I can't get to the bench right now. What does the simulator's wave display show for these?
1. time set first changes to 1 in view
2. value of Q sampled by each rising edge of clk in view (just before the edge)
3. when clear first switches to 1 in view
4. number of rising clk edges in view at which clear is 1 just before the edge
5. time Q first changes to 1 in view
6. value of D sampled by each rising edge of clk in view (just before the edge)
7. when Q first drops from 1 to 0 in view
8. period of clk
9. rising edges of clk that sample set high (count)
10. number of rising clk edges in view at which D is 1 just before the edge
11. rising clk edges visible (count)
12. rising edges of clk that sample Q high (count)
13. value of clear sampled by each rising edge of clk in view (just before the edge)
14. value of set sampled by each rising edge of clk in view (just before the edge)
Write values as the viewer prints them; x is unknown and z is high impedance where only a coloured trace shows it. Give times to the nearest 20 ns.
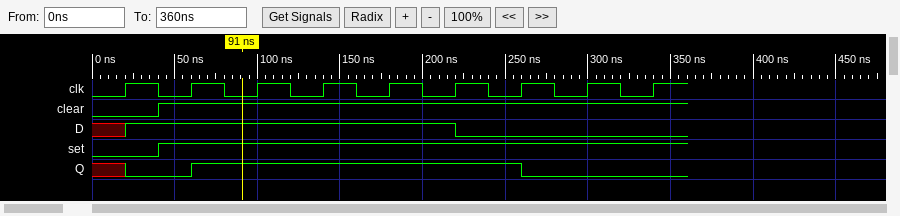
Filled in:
40 ns
x 0 1 1 1 1 1 0 0
40 ns
8
60 ns
x 1 1 1 1 1 0 0 0
260 ns
40 ns
8
5
9
5
0 1 1 1 1 1 1 1 1
0 1 1 1 1 1 1 1 1
